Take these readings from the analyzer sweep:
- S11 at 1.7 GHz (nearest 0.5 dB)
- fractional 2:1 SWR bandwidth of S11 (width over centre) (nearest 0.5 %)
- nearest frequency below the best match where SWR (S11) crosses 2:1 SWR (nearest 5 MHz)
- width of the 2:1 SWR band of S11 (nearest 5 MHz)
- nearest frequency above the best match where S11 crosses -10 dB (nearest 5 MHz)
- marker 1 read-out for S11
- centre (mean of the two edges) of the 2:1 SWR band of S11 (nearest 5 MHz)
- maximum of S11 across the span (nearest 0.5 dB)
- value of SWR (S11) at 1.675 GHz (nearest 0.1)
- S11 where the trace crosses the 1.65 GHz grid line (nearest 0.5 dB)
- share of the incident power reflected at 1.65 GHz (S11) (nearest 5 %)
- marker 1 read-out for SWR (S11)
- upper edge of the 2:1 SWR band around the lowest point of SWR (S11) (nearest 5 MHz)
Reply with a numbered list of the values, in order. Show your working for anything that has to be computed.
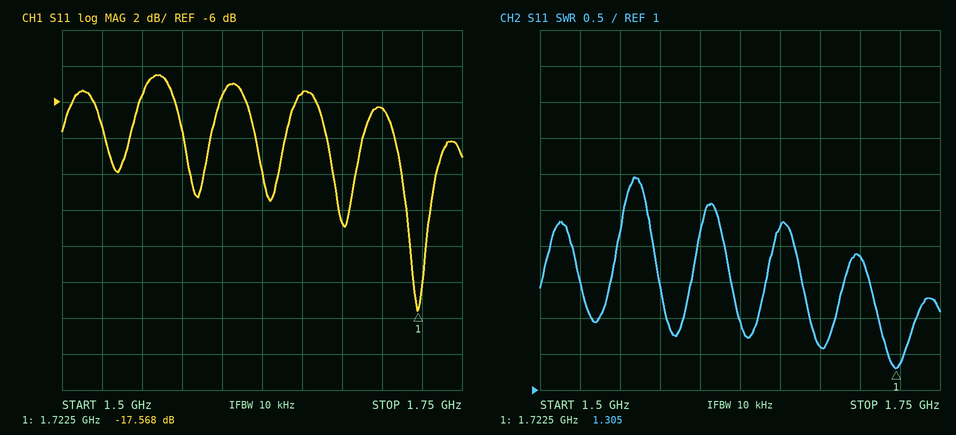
1. -6.5 dB
2. 25 MHz / 1.7225 GHz ≈ 1.5 %
3. 1.710 GHz
4. 1.735 GHz − 1.710 GHz = 25 MHz
5. 1.735 GHz
6. -17.568 dB
7. 1.725 GHz
8. -4.5 dB
9. 1.6
10. -5.5 dB
11. 10^(-5.5/10) ≈ 28.2 %, so 30 % to the nearest 5 %
12. 1.305
13. 1.735 GHz
